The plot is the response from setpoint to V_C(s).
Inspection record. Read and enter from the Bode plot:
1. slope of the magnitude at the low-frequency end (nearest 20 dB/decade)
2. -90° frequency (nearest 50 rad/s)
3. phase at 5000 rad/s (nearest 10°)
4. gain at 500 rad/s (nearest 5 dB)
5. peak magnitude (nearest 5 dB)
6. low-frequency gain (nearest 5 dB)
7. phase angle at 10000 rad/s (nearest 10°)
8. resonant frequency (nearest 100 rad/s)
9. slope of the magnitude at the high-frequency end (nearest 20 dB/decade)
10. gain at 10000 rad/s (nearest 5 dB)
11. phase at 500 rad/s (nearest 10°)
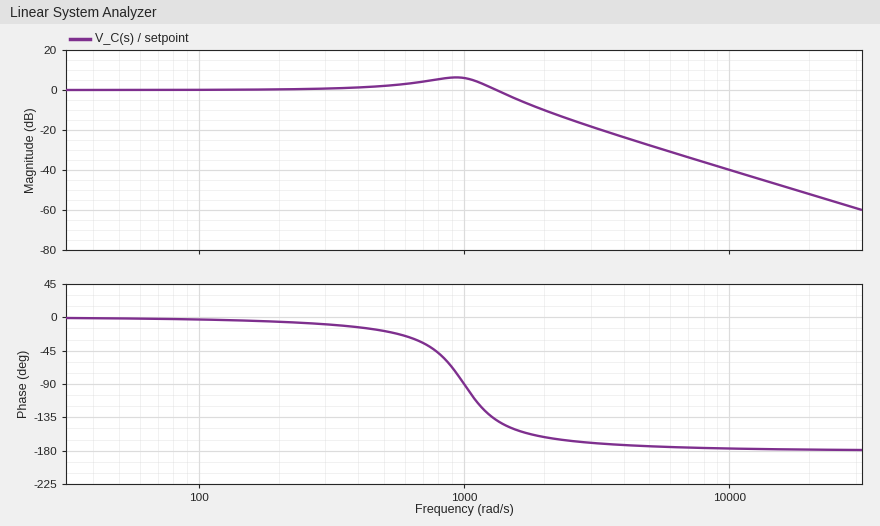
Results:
0 dB/decade
1000 rad/s
-170°
0 dB
5 dB
0 dB
-180°
900 rad/s
-40 dB/decade
-40 dB
-20°
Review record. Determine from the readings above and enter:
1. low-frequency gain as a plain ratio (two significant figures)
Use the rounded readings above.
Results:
1.0
